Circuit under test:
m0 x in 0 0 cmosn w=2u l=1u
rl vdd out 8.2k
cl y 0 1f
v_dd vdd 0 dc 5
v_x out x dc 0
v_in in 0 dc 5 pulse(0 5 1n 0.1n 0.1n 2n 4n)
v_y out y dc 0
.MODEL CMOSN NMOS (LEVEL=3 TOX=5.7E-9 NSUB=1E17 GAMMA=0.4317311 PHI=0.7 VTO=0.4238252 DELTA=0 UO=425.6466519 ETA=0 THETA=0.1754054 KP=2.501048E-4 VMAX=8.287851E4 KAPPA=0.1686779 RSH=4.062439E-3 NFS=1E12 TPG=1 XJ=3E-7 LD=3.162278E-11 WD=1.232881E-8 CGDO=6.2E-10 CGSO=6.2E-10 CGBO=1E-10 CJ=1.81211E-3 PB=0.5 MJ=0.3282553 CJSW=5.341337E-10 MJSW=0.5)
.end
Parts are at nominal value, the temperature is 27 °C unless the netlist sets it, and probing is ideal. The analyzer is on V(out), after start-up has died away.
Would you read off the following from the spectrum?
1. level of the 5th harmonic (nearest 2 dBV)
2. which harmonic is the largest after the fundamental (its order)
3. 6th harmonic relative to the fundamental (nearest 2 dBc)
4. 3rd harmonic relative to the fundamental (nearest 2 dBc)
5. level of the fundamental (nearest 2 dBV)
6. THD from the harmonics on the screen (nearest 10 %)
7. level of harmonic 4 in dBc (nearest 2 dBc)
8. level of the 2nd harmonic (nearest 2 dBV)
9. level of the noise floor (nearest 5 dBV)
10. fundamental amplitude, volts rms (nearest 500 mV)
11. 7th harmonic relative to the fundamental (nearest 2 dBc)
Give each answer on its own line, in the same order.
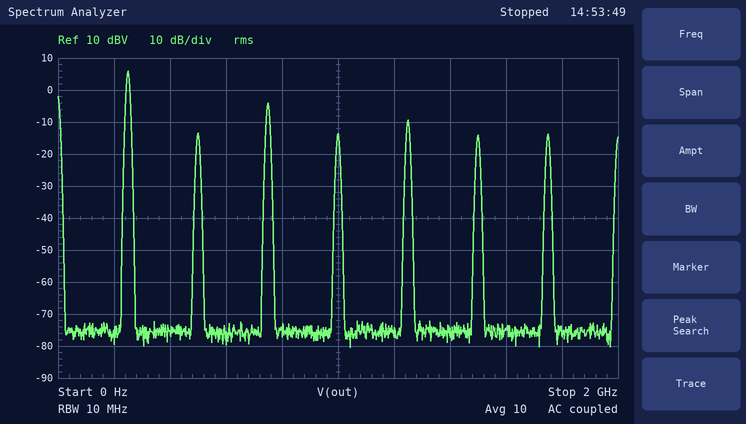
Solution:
-10 dBV
3
-20 dBc
-10 dBc
6 dBV
40 %
-20 dBc
-14 dBV
-75 dBV
2.0 V
-20 dBc
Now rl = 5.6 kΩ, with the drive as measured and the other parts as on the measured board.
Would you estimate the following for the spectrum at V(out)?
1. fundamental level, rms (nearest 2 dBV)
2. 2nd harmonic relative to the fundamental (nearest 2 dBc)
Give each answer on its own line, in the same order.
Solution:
6 dBV
-20 dBc
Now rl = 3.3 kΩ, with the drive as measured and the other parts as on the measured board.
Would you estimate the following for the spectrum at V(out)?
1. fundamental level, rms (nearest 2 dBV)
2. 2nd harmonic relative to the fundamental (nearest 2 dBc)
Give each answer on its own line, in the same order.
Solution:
4 dBV
-22 dBc
